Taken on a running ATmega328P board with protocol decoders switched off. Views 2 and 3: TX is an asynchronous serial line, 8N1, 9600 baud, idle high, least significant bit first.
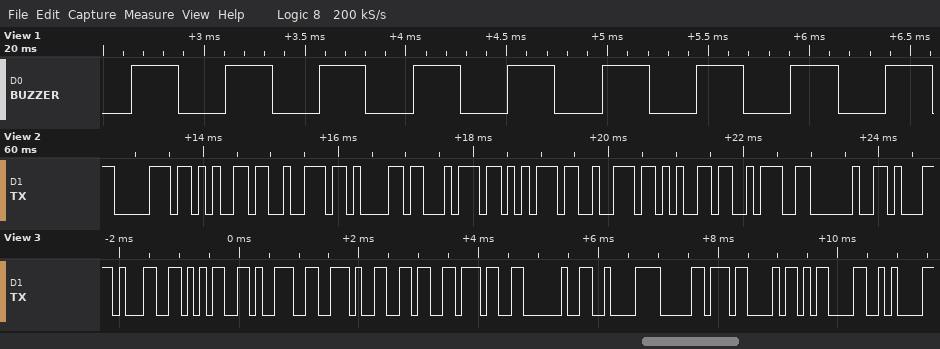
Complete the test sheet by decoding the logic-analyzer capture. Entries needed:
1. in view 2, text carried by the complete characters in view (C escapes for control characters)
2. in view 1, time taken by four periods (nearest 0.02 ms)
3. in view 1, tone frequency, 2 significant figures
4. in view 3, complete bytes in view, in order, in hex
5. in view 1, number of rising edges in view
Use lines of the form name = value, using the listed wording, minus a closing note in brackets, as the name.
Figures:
in view 2, text carried by the complete characters in view = "perature: "
in view 1, time taken by four periods = 1.88 ms
in view 1, tone frequency, 2 significant figures = 2.1 kHz
in view 3, complete bytes in view, in order, in hex = 31 35 39 2E 36 37 20 C2 B0 43 0D 0A
in view 1, number of rising edges in view = 9
